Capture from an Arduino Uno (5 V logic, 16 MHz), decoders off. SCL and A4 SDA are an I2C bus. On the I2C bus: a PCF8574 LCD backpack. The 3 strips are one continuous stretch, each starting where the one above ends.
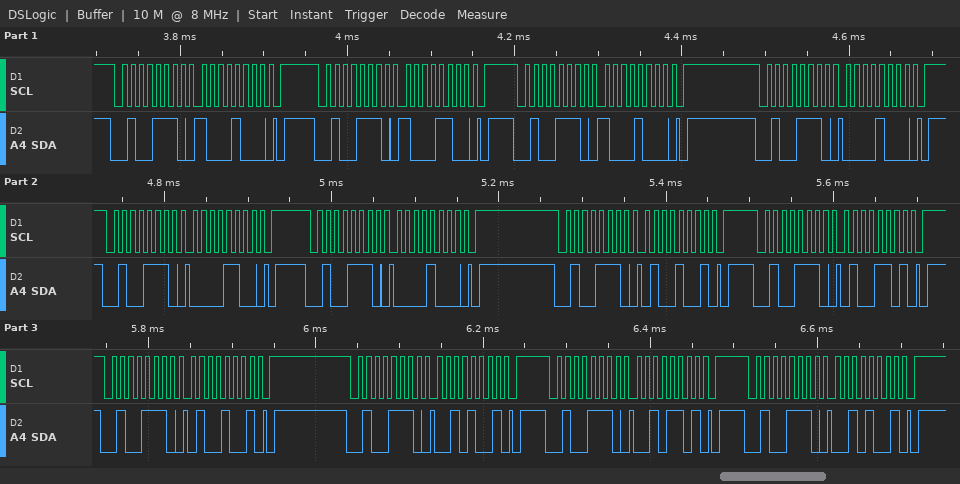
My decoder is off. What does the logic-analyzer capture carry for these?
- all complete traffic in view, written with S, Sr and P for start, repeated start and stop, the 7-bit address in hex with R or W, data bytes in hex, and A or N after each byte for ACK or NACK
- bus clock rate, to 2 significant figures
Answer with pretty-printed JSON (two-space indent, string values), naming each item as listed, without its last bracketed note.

{
  "all complete traffic in view, written with S, Sr and P for start, repeated start and stop, the 7-bit address in hex with R or W, data bytes in hex, and A or N after each byte for ACK or NACK": "S 27W A 88 A P S 27W A 8C A P S 27W A 88 A P S 27W A 08 A P S 27W A 0C A P S 27W A 08 A P S 27W A 49 A P S 27W A 4D A P S 27W A 49 A P S 27W A 29 A P S 27W A 2D A P S 27W A 29 A P",
  "bus clock rate, to 2 significant figures": "100 kHz"
}
